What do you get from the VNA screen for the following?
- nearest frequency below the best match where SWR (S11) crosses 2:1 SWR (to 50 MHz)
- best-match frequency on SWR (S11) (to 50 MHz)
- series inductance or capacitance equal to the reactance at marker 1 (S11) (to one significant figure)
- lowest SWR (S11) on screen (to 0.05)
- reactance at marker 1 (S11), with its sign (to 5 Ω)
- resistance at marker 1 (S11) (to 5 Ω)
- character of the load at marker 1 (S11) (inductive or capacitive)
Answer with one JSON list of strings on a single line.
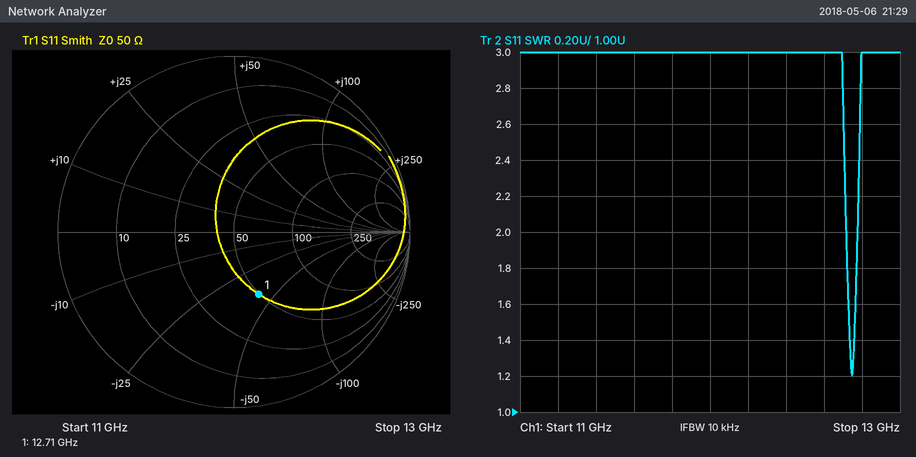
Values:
["12.70 GHz", "12.75 GHz", "300 fF", "1.20", "-40 Ω", "50 Ω", "capacitive"]
